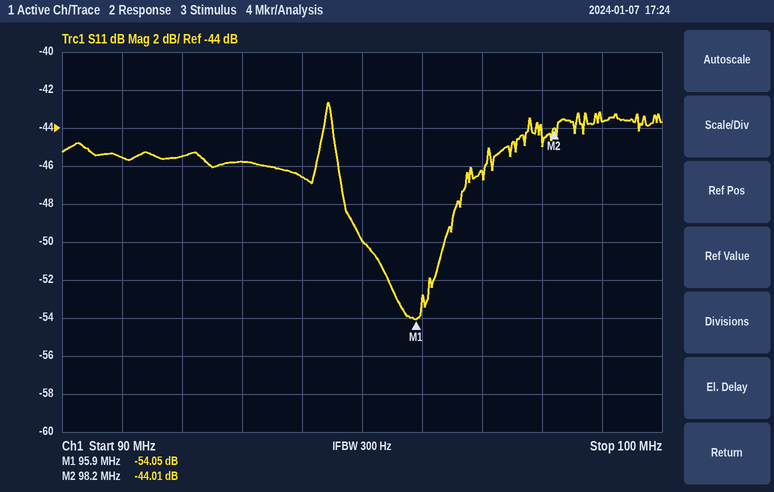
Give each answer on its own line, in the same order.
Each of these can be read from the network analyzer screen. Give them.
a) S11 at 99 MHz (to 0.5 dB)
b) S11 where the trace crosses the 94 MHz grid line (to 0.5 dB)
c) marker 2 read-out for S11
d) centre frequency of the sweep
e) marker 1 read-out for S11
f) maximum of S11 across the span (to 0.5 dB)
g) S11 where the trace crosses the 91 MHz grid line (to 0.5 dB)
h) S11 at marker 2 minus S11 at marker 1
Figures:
-43.5 dB
-46.5 dB
-44.01 dB
95 MHz
-54.05 dB
-42.5 dB
-45.5 dB
10.04 dB
